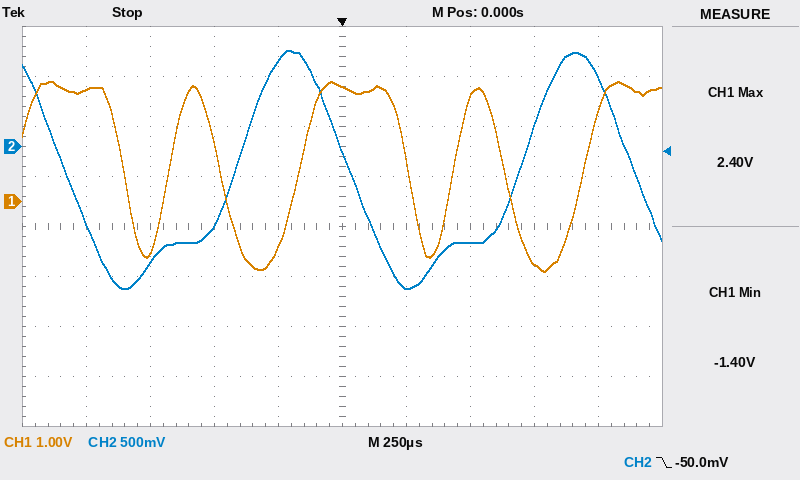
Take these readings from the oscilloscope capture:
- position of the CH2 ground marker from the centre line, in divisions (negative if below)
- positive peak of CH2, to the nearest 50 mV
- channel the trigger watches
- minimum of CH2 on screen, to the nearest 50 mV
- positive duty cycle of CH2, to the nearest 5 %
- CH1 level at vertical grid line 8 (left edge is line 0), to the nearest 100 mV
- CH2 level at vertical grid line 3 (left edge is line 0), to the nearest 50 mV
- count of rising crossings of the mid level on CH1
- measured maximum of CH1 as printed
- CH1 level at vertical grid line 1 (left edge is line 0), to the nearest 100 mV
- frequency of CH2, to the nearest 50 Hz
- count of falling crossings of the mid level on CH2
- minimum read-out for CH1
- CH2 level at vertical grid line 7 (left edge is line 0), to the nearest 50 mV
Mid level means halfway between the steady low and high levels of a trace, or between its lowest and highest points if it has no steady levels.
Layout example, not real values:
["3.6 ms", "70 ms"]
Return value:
["+1.6 div", "950 mV", "CH2", "-1.40 V", "40 %", "-1.2 V", "-800 mV", "4", "2.40 V", "2.2 V", "900 Hz", "3", "-1.40 V", "-950 mV"]
